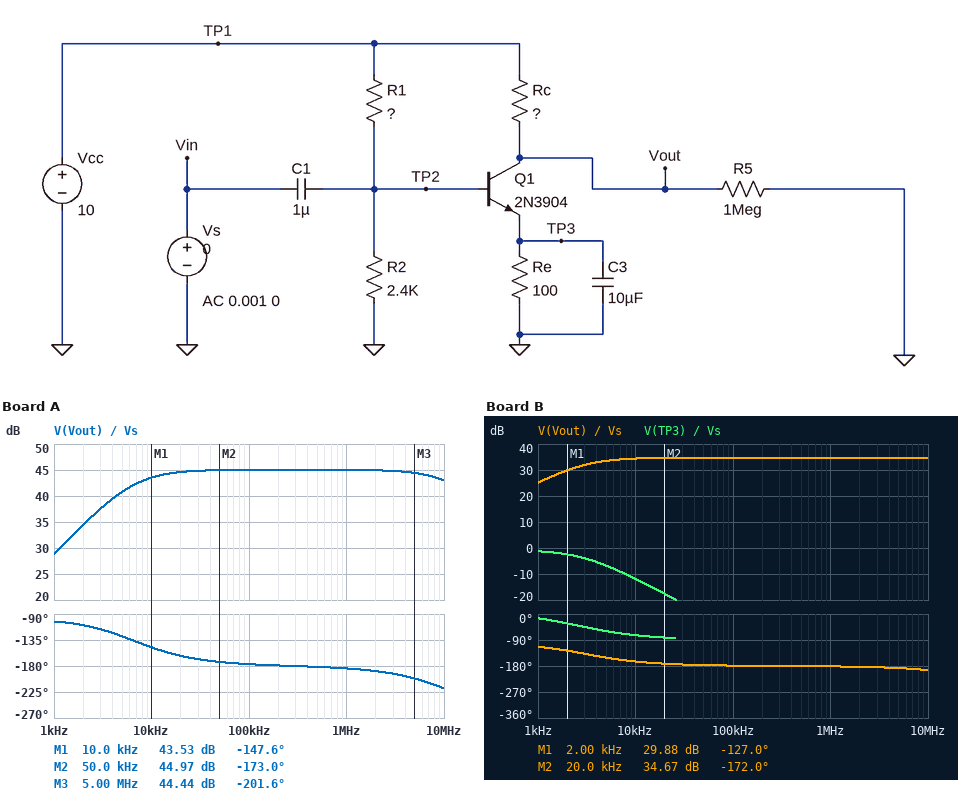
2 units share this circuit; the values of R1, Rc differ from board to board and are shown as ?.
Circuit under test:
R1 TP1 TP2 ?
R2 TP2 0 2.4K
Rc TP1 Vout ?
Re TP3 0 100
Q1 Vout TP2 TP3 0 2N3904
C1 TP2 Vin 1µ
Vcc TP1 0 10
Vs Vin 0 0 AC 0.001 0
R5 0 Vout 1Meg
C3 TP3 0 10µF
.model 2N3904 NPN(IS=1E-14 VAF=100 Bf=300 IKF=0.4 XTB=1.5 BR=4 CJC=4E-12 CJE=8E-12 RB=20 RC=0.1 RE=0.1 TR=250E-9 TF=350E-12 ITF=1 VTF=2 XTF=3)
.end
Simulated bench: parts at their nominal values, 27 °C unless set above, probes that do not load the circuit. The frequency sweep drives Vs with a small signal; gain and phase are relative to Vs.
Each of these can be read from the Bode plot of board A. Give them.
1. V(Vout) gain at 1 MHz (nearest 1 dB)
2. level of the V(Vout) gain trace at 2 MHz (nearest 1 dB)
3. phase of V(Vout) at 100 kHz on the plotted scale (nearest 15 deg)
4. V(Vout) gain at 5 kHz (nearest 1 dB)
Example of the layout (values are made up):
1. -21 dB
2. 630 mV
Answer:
1. 45 dB
2. 45 dB
3. -180 deg
4. 41 dB
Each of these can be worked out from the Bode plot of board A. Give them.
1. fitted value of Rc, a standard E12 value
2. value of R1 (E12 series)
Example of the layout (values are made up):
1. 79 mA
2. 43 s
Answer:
1. 470 Ω
2. 10 kΩ
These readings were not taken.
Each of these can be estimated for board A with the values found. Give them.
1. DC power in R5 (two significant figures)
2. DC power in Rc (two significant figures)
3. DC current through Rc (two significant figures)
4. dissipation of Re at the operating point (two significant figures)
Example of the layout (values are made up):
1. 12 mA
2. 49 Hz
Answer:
1. 22 µW
2. 61 mW
3. 11 mA
4. 13 mW
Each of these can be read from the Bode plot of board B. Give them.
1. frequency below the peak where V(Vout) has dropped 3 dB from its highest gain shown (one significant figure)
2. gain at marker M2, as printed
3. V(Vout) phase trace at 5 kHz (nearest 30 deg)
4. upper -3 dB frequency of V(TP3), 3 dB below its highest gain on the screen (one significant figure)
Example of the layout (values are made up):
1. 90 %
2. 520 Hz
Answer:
1. 3 kHz
2. 34.67 dB
3. -150 deg
4. 3 kHz
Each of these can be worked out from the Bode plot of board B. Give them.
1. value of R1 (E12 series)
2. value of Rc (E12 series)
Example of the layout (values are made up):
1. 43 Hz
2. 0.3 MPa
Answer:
1. 18 kΩ
2. 330 Ω
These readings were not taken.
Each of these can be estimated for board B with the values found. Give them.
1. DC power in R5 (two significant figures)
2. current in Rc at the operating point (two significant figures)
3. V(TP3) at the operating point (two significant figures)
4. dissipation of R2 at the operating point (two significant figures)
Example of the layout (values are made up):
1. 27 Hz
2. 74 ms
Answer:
1. 72 µW
2. 4.5 mA
3. 450 mV
4. 550 µW
